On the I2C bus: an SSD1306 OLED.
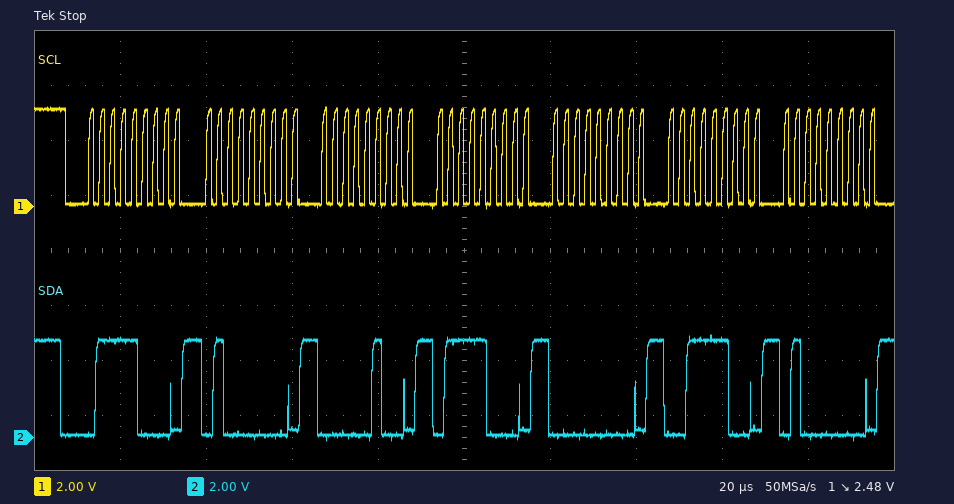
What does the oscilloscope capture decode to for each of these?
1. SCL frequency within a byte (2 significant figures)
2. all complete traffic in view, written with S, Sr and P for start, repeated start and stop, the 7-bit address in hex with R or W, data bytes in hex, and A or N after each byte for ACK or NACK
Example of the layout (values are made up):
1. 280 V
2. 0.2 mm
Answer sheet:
1. 400 kHz
2. S 3CW A 40 A 04 A 78 A 00 A 3C A 40 A
